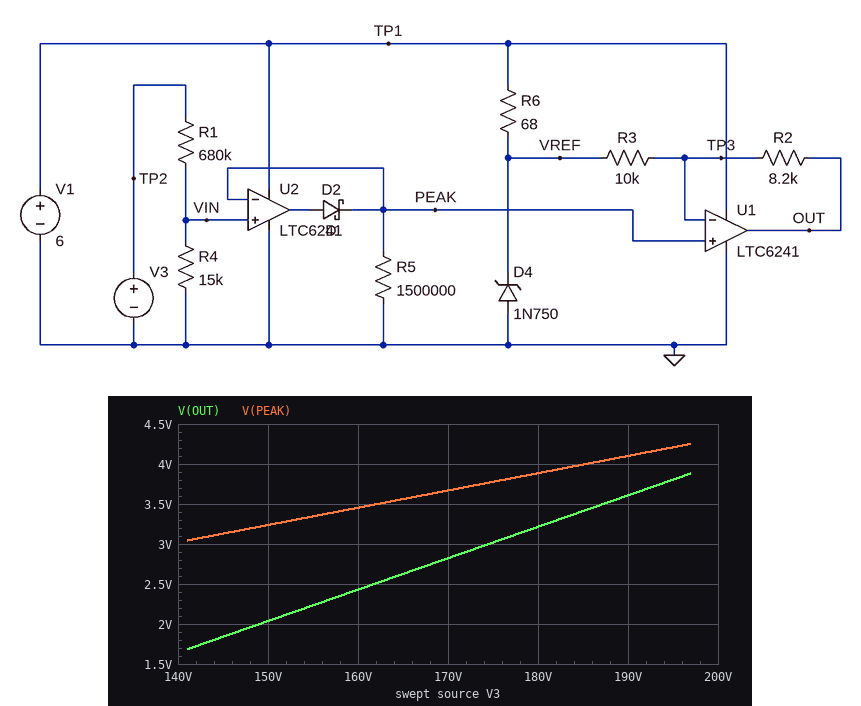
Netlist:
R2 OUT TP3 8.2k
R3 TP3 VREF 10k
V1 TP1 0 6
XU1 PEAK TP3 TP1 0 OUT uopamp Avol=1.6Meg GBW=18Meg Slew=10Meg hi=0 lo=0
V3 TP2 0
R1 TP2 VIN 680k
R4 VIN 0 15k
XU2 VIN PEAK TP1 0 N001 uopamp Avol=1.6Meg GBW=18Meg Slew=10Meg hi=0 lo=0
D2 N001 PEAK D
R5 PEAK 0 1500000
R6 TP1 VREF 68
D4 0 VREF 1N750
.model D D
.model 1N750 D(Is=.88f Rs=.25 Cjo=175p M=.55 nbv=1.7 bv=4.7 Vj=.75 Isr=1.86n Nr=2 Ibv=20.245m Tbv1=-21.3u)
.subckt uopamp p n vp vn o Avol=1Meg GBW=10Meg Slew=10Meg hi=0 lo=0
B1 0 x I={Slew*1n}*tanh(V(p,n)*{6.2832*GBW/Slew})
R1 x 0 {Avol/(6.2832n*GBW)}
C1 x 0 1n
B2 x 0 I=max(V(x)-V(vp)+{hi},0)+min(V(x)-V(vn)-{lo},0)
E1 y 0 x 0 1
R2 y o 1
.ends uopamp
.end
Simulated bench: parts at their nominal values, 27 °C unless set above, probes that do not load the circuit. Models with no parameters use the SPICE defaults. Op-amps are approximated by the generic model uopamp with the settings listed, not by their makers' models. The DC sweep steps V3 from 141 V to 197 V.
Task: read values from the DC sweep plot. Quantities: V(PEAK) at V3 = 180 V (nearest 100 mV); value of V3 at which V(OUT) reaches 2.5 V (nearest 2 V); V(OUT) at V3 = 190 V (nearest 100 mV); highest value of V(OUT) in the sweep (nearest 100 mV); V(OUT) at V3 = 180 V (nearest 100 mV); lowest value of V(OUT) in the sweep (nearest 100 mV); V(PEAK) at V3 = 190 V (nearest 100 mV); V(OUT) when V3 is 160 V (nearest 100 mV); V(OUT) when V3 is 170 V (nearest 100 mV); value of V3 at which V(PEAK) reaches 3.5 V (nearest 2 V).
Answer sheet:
3.9 V
162 V
3.6 V
3.9 V
3.2 V
1.7 V
4.1 V
2.4 V
2.8 V
162 V
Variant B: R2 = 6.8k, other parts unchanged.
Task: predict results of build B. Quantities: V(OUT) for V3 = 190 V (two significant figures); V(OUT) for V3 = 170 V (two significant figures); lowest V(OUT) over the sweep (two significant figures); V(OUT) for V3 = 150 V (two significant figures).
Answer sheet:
3.7 V
3.0 V
1.9 V
2.2 V
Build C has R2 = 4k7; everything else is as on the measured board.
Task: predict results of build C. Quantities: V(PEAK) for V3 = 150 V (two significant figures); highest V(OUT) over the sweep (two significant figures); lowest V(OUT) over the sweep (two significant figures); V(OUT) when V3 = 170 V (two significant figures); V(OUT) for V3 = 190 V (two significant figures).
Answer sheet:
3.2 V
4.0 V
2.3 V
3.2 V
3.8 V
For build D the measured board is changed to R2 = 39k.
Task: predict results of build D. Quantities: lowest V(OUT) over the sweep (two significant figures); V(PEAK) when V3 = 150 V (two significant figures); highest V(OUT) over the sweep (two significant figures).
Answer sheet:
-9.9 mV
3.2 V
2.5 V
